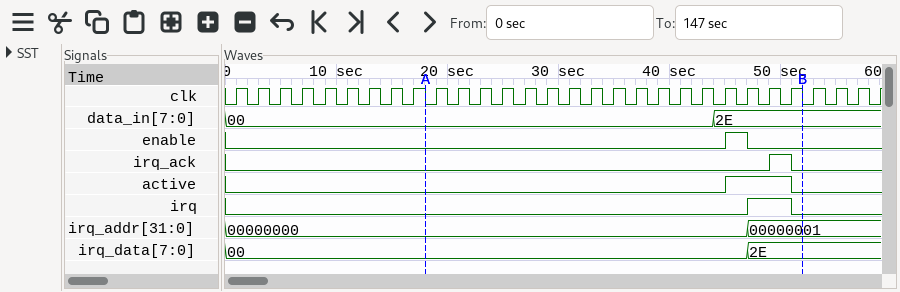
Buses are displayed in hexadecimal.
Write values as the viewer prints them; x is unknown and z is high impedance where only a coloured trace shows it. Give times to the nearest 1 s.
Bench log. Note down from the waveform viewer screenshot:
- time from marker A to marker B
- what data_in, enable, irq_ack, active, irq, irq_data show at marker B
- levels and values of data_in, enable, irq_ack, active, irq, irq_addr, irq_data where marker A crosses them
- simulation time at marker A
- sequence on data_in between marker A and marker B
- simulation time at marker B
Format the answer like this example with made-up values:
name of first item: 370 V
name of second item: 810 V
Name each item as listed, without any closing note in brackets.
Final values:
time from marker A to marker B: 34 s
what data_in, enable, irq_ack, active, irq, irq_data show at marker B: data_in=2E, enable=0, irq_ack=0, active=0, irq=0, irq_data=2E
levels and values of data_in, enable, irq_ack, active, irq, irq_addr, irq_data where marker A crosses them: data_in=00, enable=0, irq_ack=0, active=0, irq=0, irq_addr=00000000, irq_data=00
simulation time at marker A: 18 s
sequence on data_in between marker A and marker B: 00, 2E
simulation time at marker B: 52 s
